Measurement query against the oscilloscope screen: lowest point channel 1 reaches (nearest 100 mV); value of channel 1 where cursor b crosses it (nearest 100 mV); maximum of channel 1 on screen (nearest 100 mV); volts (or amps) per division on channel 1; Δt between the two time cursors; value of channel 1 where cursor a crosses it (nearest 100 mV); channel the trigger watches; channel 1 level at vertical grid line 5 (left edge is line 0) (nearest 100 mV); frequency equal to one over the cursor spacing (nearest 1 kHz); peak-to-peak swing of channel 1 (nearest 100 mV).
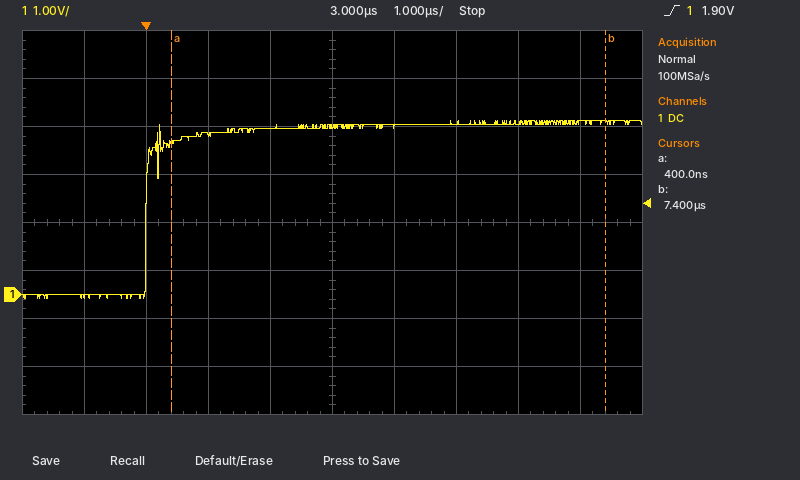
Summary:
-100 mV
3.6 V
3.6 V
1 V
7.0 µs
3.1 V
channel 1
3.5 V
143 kHz
3.7 V
